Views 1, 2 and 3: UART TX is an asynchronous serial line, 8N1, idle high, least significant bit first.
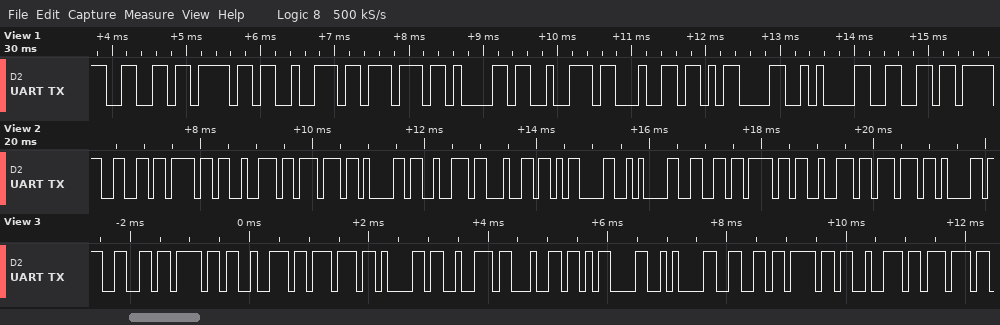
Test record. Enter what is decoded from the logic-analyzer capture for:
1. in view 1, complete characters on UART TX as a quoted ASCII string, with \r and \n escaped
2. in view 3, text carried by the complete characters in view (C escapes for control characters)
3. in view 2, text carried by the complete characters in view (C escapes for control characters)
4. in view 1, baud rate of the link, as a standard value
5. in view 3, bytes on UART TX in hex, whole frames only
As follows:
"forward\r\nf"
"forward\r\nforw"
"forward\r\nforwa"
9600 baud
66 6F 72 77 61 72 64 0D 0A 66 6F 72 77
